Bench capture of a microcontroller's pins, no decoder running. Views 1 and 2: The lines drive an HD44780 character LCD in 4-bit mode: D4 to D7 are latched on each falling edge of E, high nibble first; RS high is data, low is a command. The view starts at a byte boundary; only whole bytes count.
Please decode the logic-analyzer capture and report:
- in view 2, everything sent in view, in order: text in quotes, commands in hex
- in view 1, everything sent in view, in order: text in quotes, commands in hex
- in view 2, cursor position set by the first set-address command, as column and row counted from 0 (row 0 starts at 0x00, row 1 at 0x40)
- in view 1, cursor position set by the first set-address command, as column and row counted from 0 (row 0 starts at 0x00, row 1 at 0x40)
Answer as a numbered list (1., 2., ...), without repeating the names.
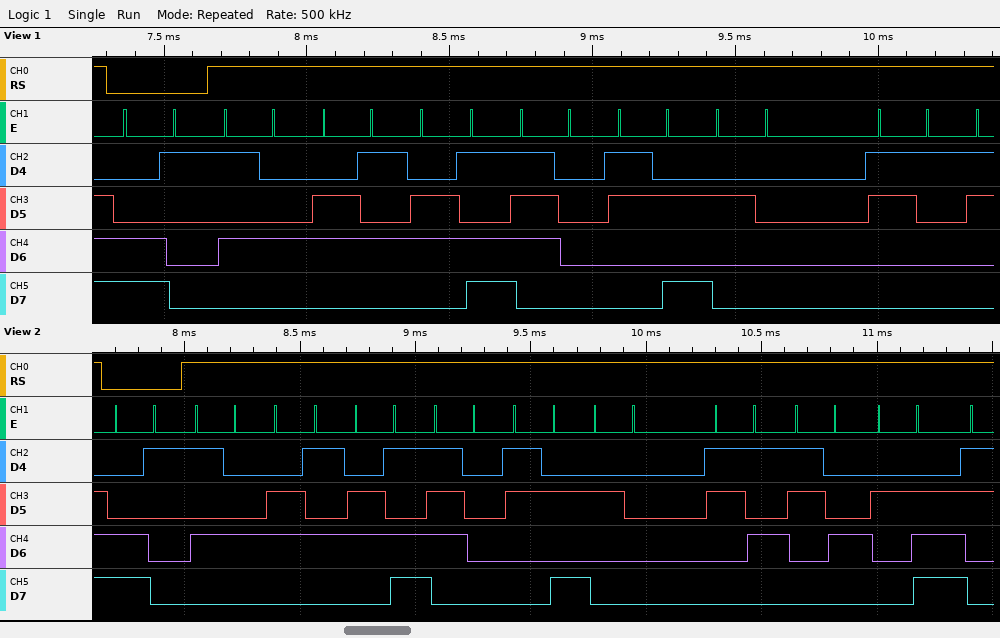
1. 0xC1 "Temp: 54."
2. 0xC1 "Temp: 1"
3. column 1, row 1
4. column 1, row 1
